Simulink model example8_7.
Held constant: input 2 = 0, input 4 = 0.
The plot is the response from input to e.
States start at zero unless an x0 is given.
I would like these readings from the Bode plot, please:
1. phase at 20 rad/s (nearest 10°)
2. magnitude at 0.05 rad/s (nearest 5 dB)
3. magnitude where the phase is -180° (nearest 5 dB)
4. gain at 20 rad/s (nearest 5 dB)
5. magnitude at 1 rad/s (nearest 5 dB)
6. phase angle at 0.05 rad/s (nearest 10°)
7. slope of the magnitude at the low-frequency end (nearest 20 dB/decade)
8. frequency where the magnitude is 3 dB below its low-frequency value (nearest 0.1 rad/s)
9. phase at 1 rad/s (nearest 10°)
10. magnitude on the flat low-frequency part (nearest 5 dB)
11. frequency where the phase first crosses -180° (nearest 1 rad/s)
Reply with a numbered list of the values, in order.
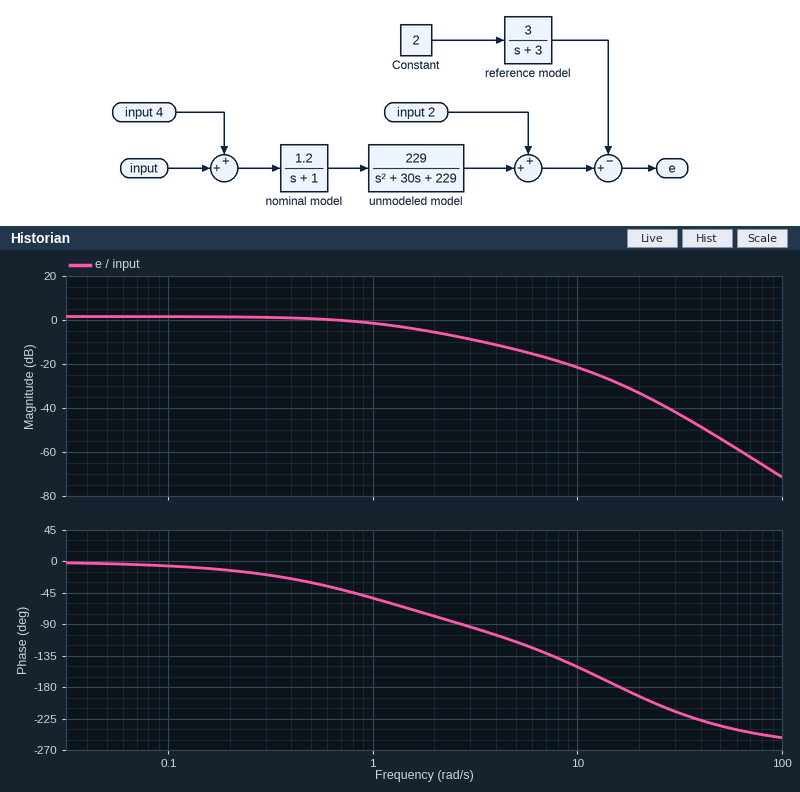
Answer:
1. -190°
2. 0 dB
3. -30 dB
4. -35 dB
5. 0 dB
6. 0°
7. 0 dB/decade
8. 1.0 rad/s
9. -50°
10. 0 dB
11. 16 rad/s
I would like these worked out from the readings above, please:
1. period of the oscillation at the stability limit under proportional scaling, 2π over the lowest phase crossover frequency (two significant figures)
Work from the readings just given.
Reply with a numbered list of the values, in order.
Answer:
1. 0.39 s
